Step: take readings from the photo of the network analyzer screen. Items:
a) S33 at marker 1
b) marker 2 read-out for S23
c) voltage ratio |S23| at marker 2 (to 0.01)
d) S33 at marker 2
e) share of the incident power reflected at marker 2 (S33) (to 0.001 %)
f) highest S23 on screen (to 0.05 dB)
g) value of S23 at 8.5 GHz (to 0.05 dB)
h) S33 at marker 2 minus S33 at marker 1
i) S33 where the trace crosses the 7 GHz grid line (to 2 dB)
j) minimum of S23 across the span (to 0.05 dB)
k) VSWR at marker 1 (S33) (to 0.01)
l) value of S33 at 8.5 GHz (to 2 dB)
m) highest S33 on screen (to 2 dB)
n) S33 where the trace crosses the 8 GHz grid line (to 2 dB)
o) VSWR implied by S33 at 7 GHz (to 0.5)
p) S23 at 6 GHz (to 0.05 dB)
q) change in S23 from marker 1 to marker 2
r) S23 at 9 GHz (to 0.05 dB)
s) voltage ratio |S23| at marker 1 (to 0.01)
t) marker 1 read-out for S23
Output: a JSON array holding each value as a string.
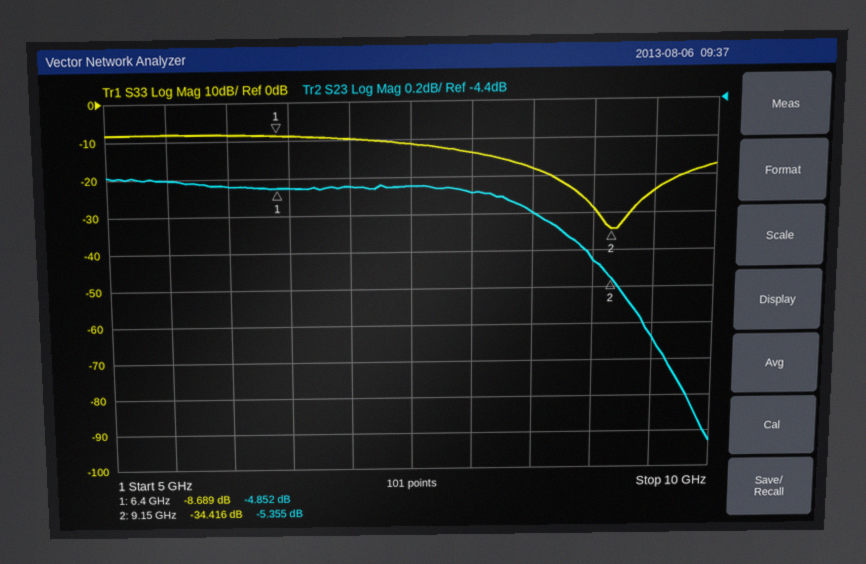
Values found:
["-8.689 dB", "-5.355 dB", "0.54", "-34.416 dB", "0.036 %", "-4.80 dB", "-5.00 dB", "-25.727 dB", "-10 dB", "-6.25 dB", "2.16", "-18 dB", "-8 dB", "-14 dB", "2.0", "-4.85 dB", "-0.503 dB", "-5.25 dB", "0.57", "-4.852 dB"]
